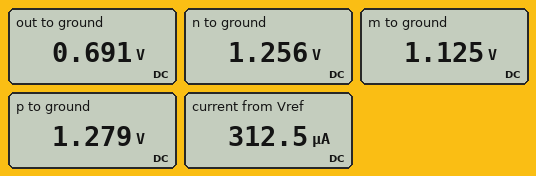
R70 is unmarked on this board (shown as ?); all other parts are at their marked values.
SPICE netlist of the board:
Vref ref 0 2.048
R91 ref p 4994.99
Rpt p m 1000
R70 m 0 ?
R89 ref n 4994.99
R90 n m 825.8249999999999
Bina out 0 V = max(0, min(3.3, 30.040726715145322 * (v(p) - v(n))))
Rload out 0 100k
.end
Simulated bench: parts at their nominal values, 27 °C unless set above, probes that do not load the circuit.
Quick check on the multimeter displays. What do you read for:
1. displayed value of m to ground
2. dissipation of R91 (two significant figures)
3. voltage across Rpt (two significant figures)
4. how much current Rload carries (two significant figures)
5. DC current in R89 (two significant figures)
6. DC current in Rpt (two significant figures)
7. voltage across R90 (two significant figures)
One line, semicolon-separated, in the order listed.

1.125 V; 120 µW; 150 mV; 6.9 µA; 160 µA; 150 µA; 130 mV
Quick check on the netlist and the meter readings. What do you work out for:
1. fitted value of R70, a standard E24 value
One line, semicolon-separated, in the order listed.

3.6 kΩ
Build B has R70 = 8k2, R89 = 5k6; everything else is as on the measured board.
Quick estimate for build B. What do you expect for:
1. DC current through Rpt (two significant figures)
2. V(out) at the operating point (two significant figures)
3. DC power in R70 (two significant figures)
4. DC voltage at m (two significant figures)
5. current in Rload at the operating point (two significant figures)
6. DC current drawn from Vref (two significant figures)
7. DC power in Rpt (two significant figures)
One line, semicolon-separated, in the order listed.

94 µA; 650 mV; 270 µW; 1.5 V; 6.5 µA; 180 µA; 8.8 µW
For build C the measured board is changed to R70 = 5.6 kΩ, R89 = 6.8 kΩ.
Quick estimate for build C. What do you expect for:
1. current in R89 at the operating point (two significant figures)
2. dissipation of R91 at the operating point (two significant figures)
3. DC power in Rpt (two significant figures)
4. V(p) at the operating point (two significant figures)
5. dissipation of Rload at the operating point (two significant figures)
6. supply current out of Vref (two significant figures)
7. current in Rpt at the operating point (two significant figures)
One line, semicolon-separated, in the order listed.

100 µA; 82 µW; 16 µW; 1.4 V; 18 µW; 230 µA; 130 µA
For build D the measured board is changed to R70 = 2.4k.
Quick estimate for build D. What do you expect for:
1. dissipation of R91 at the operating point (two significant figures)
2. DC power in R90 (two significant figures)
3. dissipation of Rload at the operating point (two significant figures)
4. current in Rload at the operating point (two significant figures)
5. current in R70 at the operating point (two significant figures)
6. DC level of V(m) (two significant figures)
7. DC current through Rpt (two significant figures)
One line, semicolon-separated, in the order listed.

180 µW; 31 µW; 7.2 µW; 8.5 µA; 380 µA; 920 mV; 190 µA
